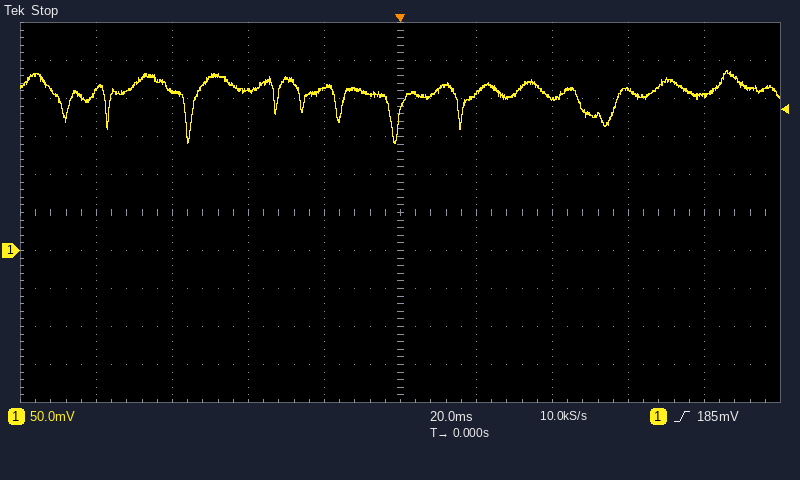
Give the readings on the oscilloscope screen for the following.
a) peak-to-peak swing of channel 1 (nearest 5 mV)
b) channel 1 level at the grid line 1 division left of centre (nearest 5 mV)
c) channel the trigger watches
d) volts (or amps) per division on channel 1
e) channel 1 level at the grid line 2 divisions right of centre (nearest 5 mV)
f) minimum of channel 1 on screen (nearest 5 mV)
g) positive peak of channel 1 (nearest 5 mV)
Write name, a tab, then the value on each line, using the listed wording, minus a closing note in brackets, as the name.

peak-to-peak swing of channel 1	95 mV
channel 1 level at the grid line 1 division left of centre	215 mV
channel the trigger watches	channel 1
volts (or amps) per division on channel 1	50 mV
channel 1 level at the grid line 2 divisions right of centre	200 mV
minimum of channel 1 on screen	140 mV
positive peak of channel 1	235 mV
